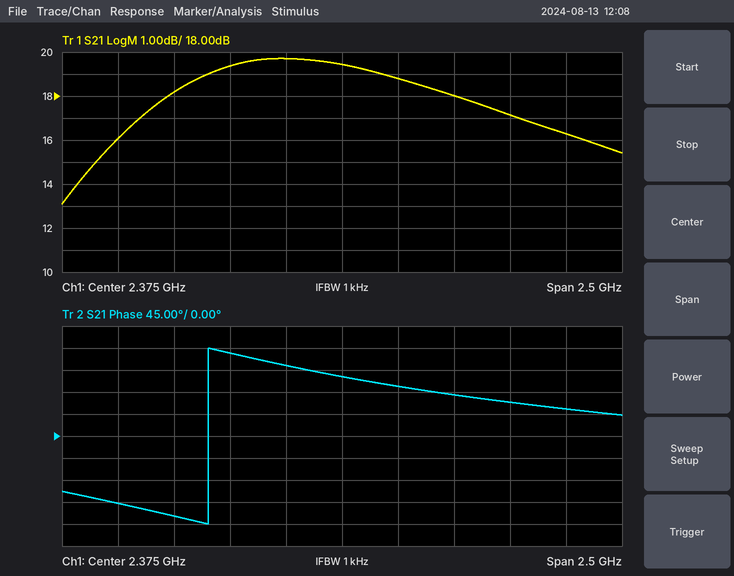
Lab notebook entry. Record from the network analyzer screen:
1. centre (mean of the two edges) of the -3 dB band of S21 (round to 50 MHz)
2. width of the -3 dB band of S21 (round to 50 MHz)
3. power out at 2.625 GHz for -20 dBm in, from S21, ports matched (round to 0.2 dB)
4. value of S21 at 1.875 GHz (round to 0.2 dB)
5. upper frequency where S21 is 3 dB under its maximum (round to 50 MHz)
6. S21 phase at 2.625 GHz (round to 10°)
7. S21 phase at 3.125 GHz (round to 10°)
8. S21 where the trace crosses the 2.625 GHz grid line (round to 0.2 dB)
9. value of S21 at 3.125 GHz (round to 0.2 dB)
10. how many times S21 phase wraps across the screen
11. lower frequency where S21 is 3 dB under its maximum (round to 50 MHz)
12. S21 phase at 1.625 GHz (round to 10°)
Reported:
2.35 GHz
1.80 GHz
-1.2 dBm
19.4 dB
3.25 GHz
100°
70°
18.8 dB
17.2 dB
1
1.45 GHz
-160°
